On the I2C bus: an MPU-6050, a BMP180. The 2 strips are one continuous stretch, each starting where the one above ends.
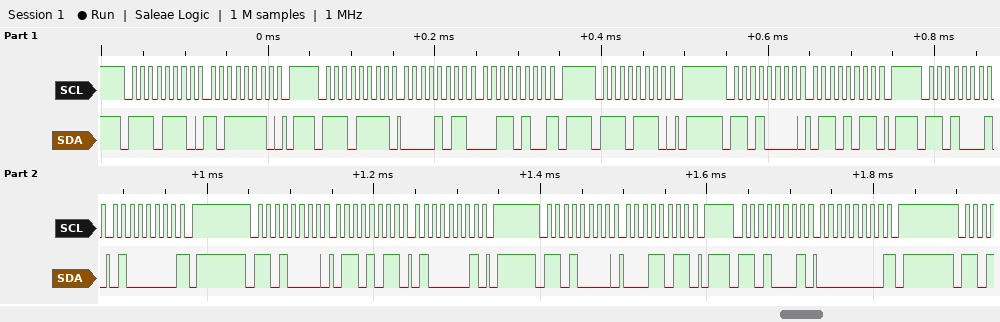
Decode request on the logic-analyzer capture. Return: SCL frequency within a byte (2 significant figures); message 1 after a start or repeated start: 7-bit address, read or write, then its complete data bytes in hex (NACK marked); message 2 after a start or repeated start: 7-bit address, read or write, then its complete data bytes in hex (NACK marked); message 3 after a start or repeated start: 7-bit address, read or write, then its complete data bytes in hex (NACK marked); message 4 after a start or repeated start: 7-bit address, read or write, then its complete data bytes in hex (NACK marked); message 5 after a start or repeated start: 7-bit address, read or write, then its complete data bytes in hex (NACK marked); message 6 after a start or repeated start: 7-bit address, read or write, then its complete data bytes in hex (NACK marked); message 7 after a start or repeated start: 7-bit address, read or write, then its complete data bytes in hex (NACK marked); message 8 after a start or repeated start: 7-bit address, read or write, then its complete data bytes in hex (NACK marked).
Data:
100 kHz
0x77 write: BE
0x77 read: 0B 34 NACK
0x77 write
0x68 write: 6B
0x68 read: 40 NACK
0x68 write: 6B 41
0x68 write: 1B
0x68 read: 00 NACK
